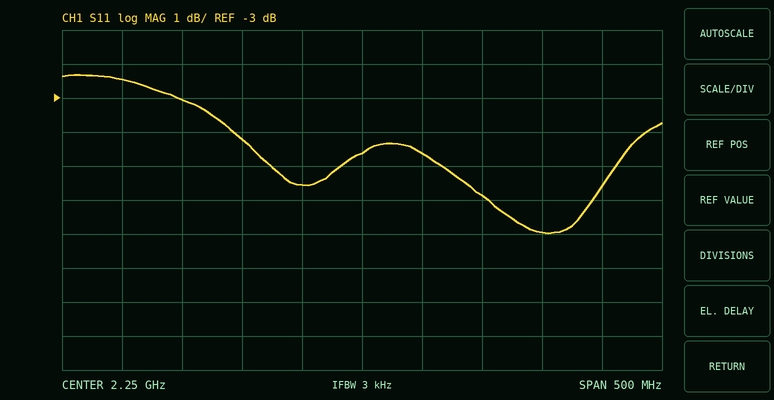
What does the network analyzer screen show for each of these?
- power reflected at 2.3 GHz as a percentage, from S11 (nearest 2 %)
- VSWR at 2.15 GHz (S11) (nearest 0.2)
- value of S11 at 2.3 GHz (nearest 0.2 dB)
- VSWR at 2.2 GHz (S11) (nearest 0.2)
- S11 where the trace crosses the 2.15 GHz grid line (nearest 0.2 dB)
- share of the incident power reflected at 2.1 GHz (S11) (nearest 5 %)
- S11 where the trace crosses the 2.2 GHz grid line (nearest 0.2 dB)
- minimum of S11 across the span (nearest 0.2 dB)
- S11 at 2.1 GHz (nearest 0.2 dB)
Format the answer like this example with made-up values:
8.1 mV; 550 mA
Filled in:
34 %; 4.2; -4.6 dB; 3.2; -4.2 dB; 50 %; -5.6 dB; -7.0 dB; -3.0 dB
